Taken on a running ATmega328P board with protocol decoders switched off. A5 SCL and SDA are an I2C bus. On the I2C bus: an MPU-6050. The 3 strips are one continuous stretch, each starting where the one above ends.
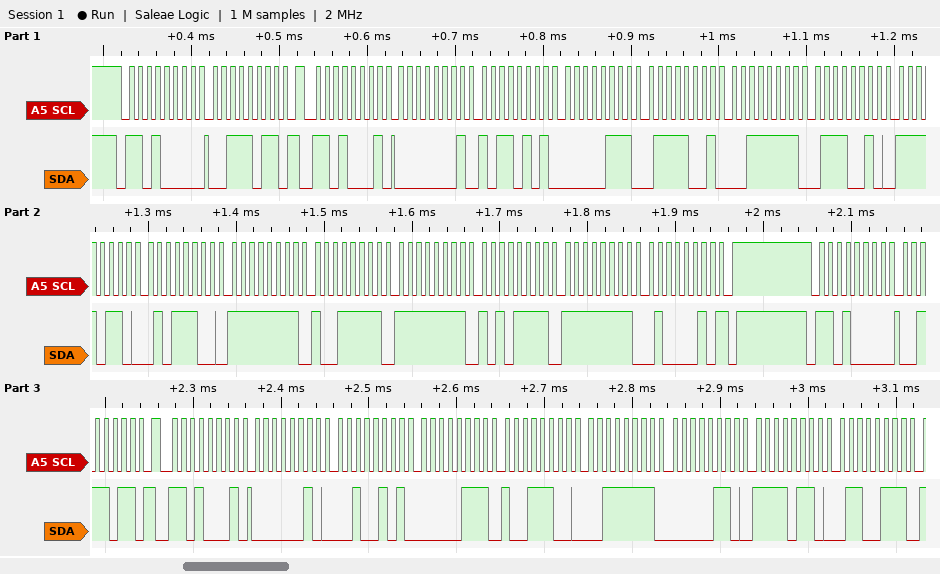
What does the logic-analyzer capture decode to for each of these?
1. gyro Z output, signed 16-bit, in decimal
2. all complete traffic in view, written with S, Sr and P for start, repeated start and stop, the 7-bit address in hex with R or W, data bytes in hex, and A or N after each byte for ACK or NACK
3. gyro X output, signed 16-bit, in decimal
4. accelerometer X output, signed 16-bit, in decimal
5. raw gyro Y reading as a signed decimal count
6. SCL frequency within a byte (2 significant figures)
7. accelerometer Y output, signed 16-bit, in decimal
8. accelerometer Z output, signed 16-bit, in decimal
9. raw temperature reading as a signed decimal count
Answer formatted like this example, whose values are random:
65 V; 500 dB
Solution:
-190; S 68W A 3B A Sr 68R A 01 A B5 A 07 A 79 A 3F A 72 A F6 A 5C A FF A 9F A FF A AF A FF A 42 N P S 68W A 3B A Sr 68R A 02 A 25 A 07 A 9C A 3F A 06 A F6 A 67 A; -97; 437; -81; 100 kHz; 1913; 16242; -2468
